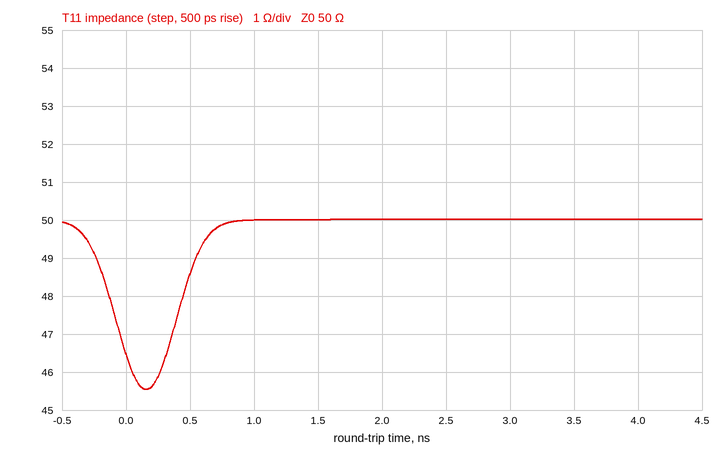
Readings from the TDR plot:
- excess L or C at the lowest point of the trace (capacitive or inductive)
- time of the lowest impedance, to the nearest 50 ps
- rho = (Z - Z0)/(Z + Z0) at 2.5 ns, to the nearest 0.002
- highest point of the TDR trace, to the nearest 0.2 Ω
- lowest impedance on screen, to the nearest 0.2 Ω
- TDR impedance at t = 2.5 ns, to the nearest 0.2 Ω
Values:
capacitive
150 ps
0.000
50.0 Ω
45.6 Ω
50.0 Ω
